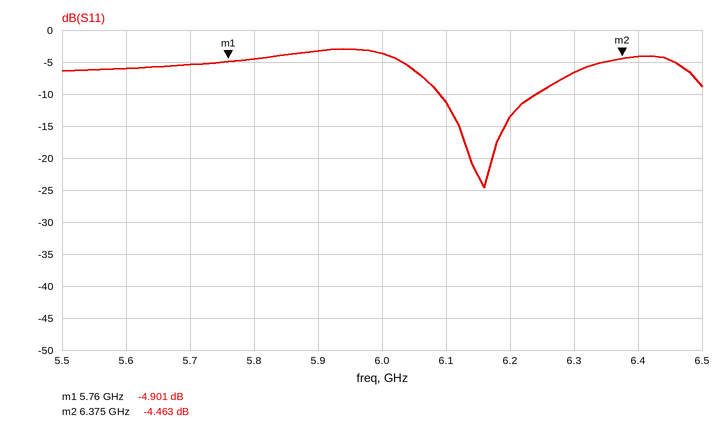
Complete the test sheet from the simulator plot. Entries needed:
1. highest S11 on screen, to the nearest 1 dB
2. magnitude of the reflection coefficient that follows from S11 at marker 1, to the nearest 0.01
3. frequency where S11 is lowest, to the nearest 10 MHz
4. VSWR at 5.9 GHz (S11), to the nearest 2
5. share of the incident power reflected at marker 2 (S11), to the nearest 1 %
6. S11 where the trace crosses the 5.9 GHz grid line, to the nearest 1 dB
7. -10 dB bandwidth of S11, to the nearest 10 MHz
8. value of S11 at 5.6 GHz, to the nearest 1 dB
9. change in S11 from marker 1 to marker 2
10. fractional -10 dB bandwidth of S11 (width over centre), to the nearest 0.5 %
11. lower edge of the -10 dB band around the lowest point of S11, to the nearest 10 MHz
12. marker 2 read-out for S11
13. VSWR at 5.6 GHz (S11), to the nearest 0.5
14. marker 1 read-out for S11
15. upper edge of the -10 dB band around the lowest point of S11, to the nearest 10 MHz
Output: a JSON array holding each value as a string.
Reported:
["-3 dB", "0.57", "6.16 GHz", "6", "36 %", "-3 dB", "150 MHz", "-6 dB", "0.438 dB", "2.5 %", "6.09 GHz", "-4.463 dB", "3.0", "-4.901 dB", "6.24 GHz"]
